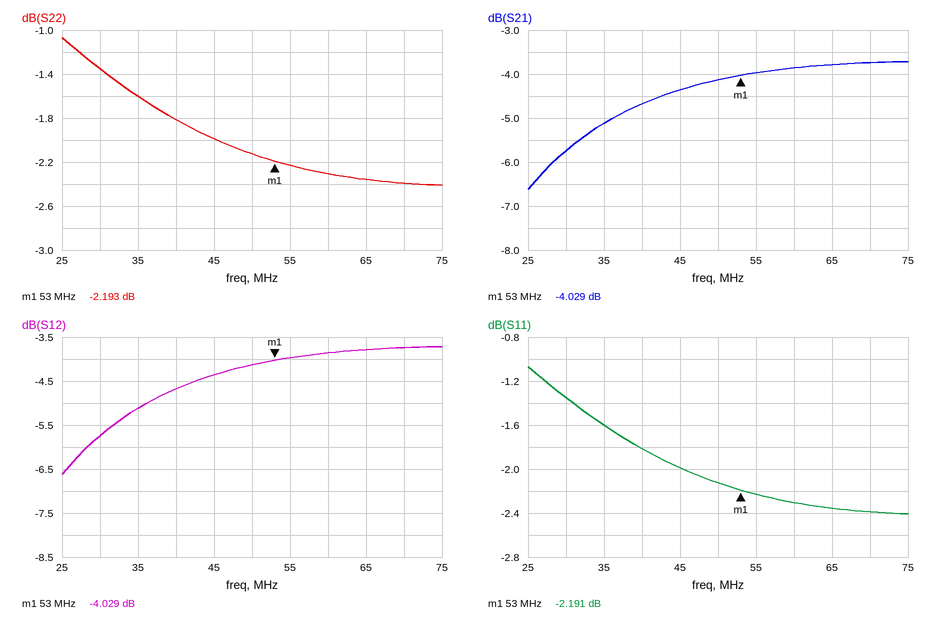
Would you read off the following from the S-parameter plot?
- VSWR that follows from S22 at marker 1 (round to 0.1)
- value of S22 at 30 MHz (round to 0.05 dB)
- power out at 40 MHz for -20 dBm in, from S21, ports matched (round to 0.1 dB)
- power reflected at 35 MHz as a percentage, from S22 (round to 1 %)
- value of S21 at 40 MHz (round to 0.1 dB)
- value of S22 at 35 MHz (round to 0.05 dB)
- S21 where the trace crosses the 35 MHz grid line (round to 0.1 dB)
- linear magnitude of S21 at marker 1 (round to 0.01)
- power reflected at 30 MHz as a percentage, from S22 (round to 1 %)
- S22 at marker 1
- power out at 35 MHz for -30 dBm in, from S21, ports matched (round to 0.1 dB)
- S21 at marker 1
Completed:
8.0
-1.35 dB
-24.7 dBm
69 %
-4.7 dB
-1.60 dB
-5.1 dB
0.63
73 %
-2.193 dB
-35.1 dBm
-4.029 dB
